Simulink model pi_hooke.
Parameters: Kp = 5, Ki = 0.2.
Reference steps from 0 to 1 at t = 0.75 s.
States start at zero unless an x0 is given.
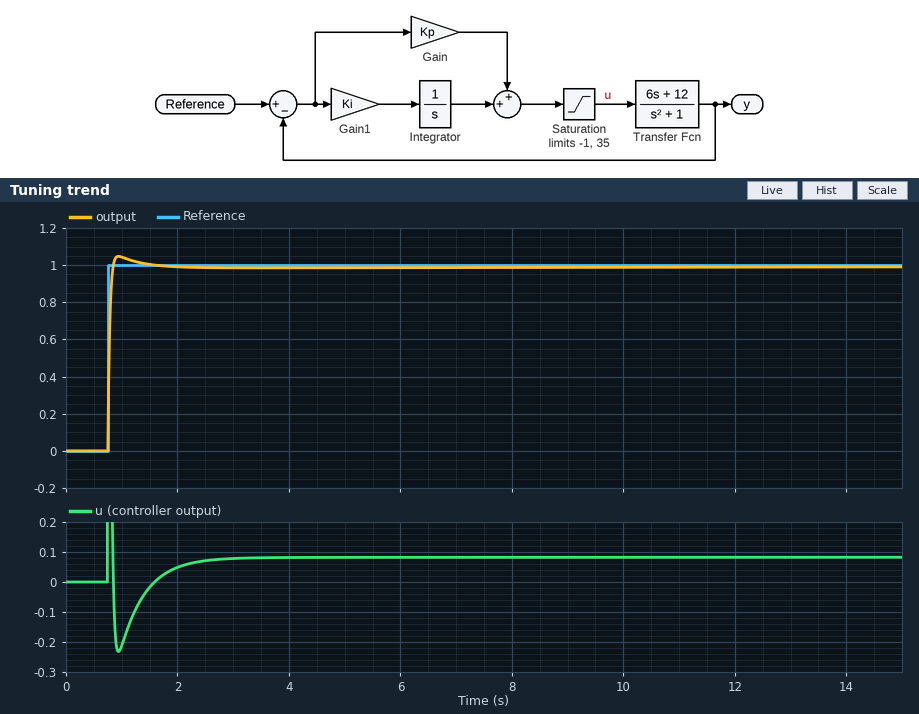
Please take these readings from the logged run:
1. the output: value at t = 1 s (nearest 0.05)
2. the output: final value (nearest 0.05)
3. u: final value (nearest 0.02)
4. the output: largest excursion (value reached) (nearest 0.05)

1.05
1.00
0.08
1.05
